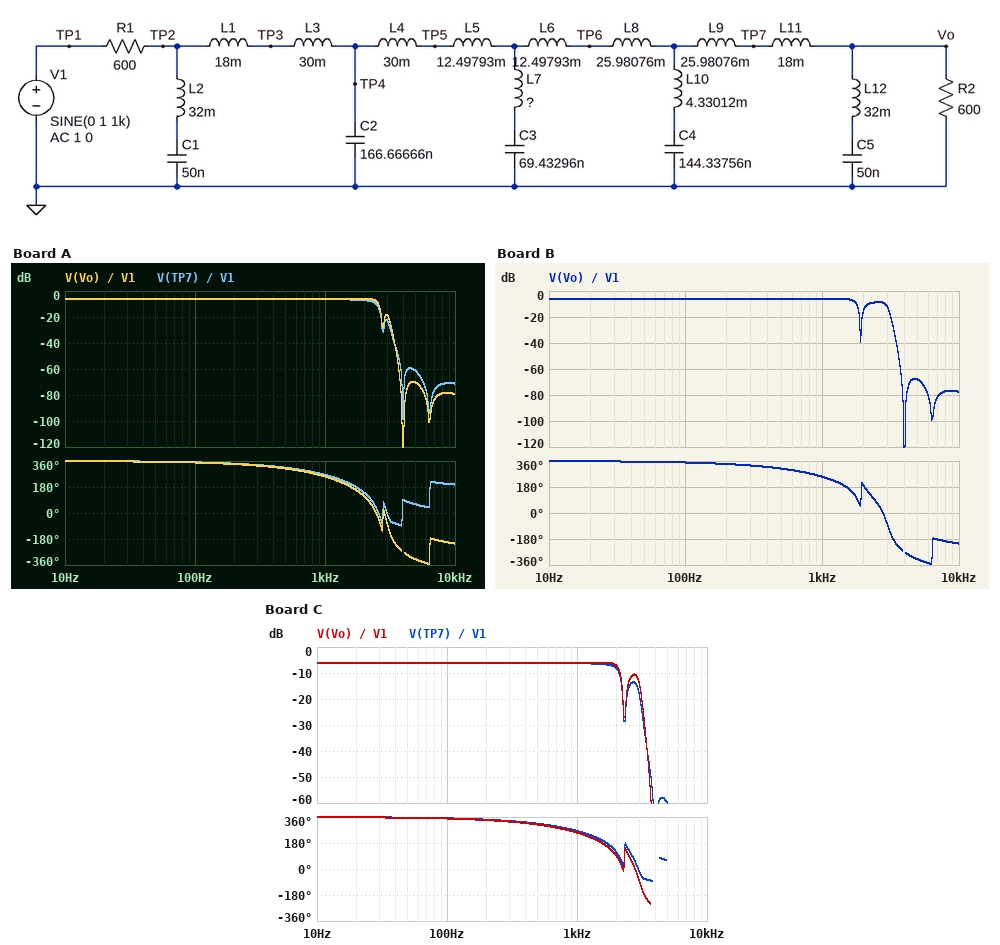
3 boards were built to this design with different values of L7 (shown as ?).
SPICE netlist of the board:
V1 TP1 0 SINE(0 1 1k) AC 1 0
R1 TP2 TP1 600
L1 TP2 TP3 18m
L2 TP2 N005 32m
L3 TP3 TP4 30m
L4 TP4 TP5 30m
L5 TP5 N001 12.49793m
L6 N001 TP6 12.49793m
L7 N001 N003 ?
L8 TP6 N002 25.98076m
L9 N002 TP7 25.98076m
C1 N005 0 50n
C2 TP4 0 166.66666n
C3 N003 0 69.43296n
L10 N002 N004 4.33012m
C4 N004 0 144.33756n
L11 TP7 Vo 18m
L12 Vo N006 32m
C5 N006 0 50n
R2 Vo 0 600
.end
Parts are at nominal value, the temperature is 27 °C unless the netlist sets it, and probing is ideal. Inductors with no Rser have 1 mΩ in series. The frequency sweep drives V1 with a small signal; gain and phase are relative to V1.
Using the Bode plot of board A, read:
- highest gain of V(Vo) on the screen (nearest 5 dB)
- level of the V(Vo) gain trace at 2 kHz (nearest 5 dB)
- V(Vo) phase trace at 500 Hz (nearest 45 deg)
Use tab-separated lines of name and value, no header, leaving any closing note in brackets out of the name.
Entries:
highest gain of V(Vo) on the screen	-5 dB
level of the V(Vo) gain trace at 2 kHz	-5 dB
V(Vo) phase trace at 500 Hz	315 deg
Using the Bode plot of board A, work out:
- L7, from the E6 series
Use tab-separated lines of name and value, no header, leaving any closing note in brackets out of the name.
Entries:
L7, from the E6 series	47 mH
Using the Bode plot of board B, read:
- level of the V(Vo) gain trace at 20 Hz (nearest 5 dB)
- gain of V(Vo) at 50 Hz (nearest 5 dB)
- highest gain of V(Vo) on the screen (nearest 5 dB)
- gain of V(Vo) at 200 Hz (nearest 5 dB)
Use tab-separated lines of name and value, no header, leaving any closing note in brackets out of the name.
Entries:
level of the V(Vo) gain trace at 20 Hz	-5 dB
gain of V(Vo) at 50 Hz	-5 dB
highest gain of V(Vo) on the screen	-5 dB
gain of V(Vo) at 200 Hz	-5 dB
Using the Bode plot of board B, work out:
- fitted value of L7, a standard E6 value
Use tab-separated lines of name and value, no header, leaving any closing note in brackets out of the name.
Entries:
fitted value of L7, a standard E6 value	100 mH
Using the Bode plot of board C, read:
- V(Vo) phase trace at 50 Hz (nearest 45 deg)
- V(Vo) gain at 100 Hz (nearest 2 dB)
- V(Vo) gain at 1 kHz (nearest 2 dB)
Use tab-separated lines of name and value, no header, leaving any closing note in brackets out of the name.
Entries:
V(Vo) phase trace at 50 Hz	360 deg
V(Vo) gain at 100 Hz	-6 dB
V(Vo) gain at 1 kHz	-6 dB
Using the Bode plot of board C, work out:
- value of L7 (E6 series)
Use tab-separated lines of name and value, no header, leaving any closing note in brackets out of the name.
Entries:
value of L7	68 mH
